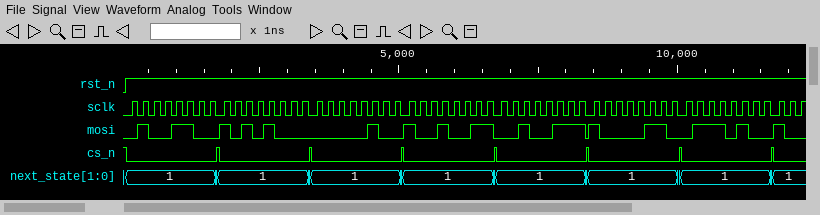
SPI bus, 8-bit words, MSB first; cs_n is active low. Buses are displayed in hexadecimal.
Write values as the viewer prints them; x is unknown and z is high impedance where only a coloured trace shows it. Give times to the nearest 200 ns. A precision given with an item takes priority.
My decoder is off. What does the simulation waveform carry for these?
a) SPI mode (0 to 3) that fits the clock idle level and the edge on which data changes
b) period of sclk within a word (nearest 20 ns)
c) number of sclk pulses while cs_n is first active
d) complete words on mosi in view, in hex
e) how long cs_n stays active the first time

0
200 ns
8
4C, A8, 04, 93, 27, 86, 74
1600 ns
